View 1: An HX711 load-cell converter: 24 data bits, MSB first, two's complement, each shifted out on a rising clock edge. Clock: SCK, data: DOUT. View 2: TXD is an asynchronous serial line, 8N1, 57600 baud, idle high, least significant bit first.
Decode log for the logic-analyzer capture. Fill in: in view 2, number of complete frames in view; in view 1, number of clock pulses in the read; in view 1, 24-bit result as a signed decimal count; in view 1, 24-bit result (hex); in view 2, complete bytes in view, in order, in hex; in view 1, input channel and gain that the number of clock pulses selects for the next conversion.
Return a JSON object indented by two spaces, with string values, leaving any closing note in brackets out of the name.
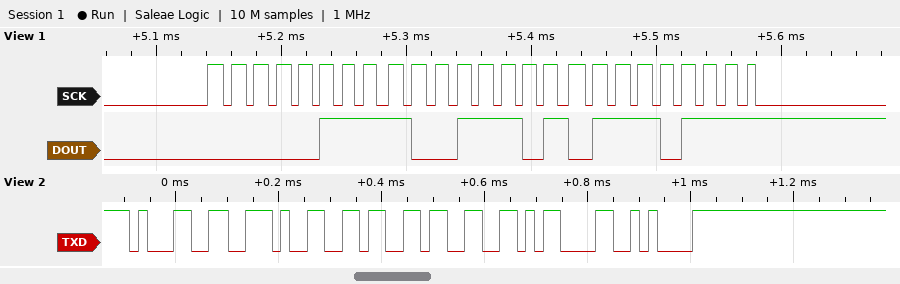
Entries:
{
  "in view 2, number of complete frames in view": "6",
  "in view 1, number of clock pulses in the read": "25",
  "in view 1, 24-bit result as a signed decimal count": "499063",
  "in view 1, 24-bit result": "0x079D77",
  "in view 2, complete bytes in view, in order, in hex": "31 2E 36 33 0D 0A",
  "in view 1, input channel and gain that the number of clock pulses selects for the next conversion": "channel A, gain 128"
}
